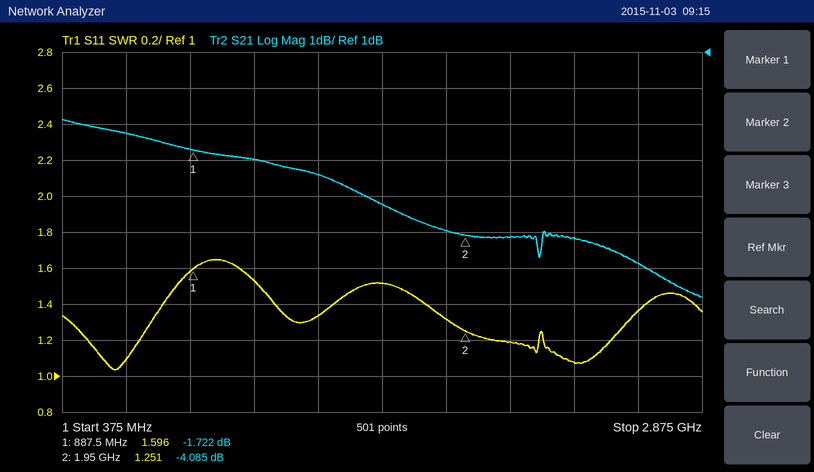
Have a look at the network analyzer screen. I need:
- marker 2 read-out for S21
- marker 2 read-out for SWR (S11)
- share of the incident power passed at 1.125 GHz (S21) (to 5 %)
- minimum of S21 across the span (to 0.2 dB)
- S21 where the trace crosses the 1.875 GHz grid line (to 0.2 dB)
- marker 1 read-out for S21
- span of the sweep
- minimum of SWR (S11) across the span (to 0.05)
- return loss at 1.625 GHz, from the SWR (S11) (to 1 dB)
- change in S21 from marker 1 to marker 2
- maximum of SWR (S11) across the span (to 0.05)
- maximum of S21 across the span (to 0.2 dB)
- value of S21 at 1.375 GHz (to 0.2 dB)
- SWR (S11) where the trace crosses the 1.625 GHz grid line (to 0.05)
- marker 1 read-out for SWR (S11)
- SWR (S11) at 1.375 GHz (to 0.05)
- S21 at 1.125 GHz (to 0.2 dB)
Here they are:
-4.085 dB
1.251
65 %
-5.8 dB
-4.0 dB
-1.722 dB
2.5 GHz
1.05
14 dB
-2.363 dB
1.65
-0.8 dB
-2.4 dB
1.50
1.596
1.35
-2.0 dB
